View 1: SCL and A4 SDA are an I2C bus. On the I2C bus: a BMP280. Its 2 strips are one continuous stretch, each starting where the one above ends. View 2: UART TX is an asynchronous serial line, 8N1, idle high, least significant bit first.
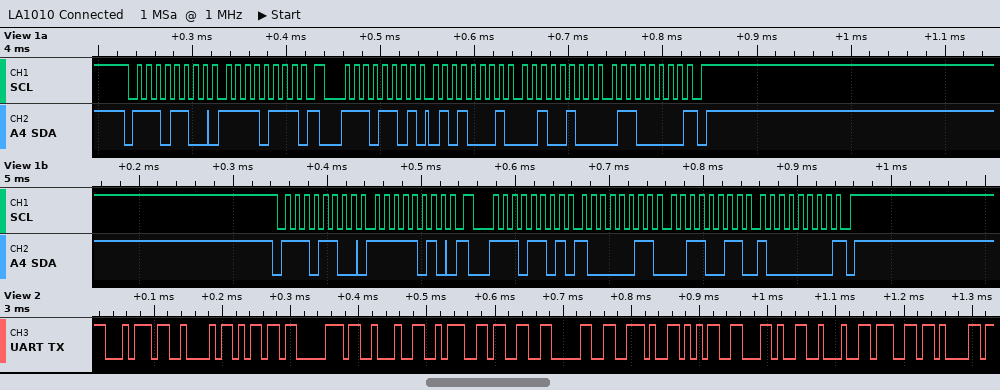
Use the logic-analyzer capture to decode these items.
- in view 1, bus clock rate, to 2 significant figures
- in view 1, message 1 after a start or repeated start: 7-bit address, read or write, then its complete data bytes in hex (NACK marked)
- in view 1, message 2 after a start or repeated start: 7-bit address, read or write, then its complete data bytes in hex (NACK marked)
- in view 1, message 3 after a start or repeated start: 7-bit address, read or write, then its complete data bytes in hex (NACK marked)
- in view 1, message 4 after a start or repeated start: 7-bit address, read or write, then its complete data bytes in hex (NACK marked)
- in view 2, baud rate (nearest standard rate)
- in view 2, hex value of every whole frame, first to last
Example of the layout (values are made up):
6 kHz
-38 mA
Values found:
100 kHz
0x76 write: F7
0x76 read: 51 24 60 NACK
0x76 write: FA
0x76 read: 83 33 80 NACK
115200 baud
0x74 0x42 0x6D 0x70 0x22 0x3A 0x33 0x30 0x2E 0x35 0x2C 0x22 0x67 0x61
